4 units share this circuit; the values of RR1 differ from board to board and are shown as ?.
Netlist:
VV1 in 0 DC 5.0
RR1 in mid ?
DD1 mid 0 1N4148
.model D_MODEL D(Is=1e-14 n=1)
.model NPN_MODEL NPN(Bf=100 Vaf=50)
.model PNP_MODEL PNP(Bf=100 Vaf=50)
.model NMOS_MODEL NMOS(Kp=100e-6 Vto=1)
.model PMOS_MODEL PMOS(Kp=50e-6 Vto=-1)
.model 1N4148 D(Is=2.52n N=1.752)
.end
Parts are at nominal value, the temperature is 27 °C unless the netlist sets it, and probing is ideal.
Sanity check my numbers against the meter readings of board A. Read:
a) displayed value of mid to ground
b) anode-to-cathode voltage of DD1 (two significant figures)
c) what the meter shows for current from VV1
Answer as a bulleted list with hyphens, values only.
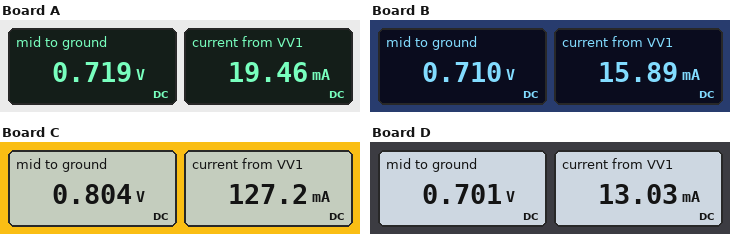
- 0.719 V
- 720 mV
- 19.46 mA
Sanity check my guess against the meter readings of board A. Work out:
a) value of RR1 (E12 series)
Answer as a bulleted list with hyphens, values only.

- 220 Ω
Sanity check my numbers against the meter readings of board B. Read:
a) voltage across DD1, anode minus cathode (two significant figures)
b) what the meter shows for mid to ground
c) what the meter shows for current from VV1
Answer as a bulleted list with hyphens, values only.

- 710 mV
- 0.710 V
- 15.89 mA
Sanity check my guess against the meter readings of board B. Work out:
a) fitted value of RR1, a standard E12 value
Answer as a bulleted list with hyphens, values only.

- 270 Ω
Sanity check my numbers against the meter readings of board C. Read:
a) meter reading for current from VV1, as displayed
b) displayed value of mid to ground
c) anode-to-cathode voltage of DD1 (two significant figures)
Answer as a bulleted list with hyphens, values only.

- 127.2 mA
- 0.804 V
- 800 mV
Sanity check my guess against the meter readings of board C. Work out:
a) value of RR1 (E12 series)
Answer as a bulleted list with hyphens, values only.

- 33 Ω
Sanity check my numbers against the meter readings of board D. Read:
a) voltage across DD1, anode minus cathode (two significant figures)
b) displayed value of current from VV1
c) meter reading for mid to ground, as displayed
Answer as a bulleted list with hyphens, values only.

- 700 mV
- 13.03 mA
- 0.701 V
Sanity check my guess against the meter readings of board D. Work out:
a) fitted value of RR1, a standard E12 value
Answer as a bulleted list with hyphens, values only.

- 330 Ω
